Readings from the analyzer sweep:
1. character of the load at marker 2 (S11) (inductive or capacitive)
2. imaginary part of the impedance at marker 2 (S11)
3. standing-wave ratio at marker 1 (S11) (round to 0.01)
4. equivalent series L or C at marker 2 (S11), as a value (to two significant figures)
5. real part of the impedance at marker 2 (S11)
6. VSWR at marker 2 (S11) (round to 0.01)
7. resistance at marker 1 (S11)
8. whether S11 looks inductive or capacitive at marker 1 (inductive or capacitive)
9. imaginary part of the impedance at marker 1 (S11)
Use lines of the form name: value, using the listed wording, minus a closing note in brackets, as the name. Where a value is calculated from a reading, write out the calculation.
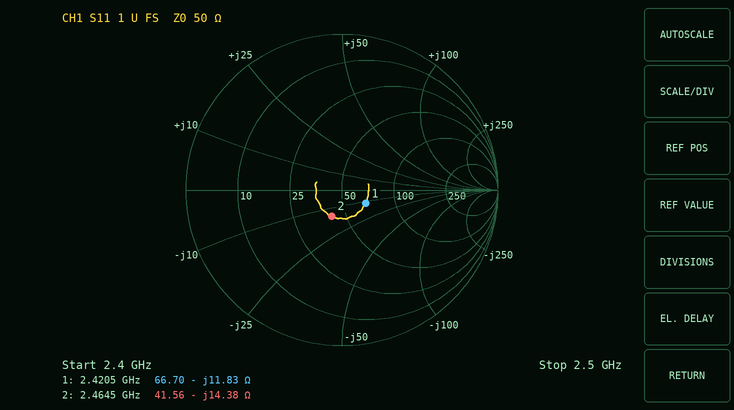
character of the load at marker 2 (S11): capacitive
imaginary part of the impedance at marker 2: -14.38 Ω
standing-wave ratio at marker 1 (S11): 1.42
equivalent series L or C at marker 2 (S11), as a value: C = 1/(2π × 2.4645 GHz × 14.38 Ω) ≈ 4.5 pF
real part of the impedance at marker 2: 41.56 Ω
VSWR at marker 2 (S11): 1.44
resistance at marker 1: 66.70 Ω
whether S11 looks inductive or capacitive at marker 1: capacitive
imaginary part of the impedance at marker 1: -11.83 Ω
